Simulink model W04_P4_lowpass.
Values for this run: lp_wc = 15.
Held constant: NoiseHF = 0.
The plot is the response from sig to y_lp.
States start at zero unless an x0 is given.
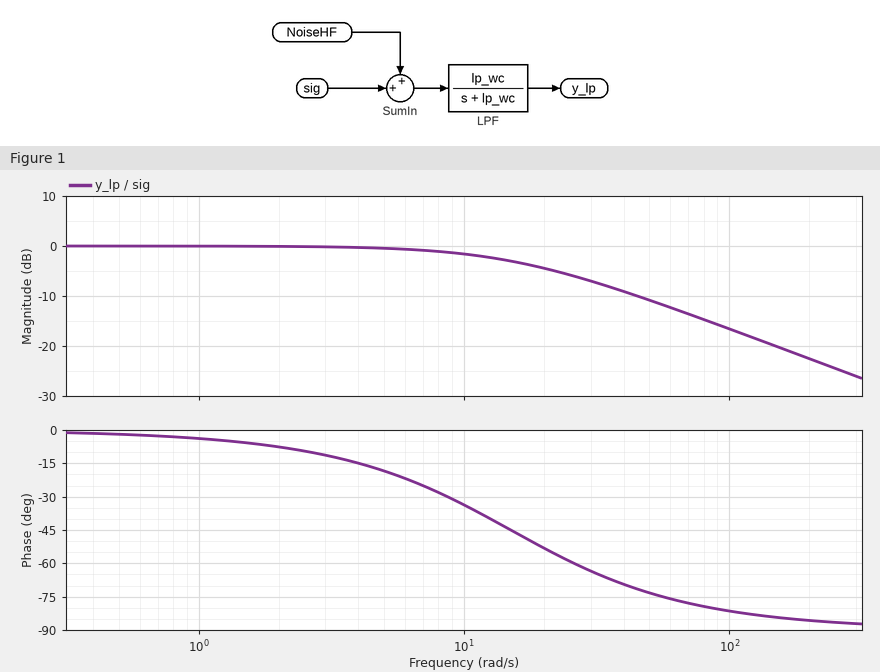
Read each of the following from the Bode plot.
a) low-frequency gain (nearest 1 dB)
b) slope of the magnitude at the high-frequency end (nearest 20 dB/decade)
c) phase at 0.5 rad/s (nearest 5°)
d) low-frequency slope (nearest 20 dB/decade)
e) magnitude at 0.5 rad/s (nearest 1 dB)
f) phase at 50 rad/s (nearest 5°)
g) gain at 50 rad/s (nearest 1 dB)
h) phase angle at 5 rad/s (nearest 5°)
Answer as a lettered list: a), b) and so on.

a) 0 dB
b) -20 dB/decade
c) 0°
d) 0 dB/decade
e) 0 dB
f) -75°
g) -11 dB
h) -20°
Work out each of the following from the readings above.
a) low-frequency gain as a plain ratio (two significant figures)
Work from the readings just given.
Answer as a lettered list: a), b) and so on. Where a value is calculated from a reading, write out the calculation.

a) 10^(0 / 20) = 1.0
